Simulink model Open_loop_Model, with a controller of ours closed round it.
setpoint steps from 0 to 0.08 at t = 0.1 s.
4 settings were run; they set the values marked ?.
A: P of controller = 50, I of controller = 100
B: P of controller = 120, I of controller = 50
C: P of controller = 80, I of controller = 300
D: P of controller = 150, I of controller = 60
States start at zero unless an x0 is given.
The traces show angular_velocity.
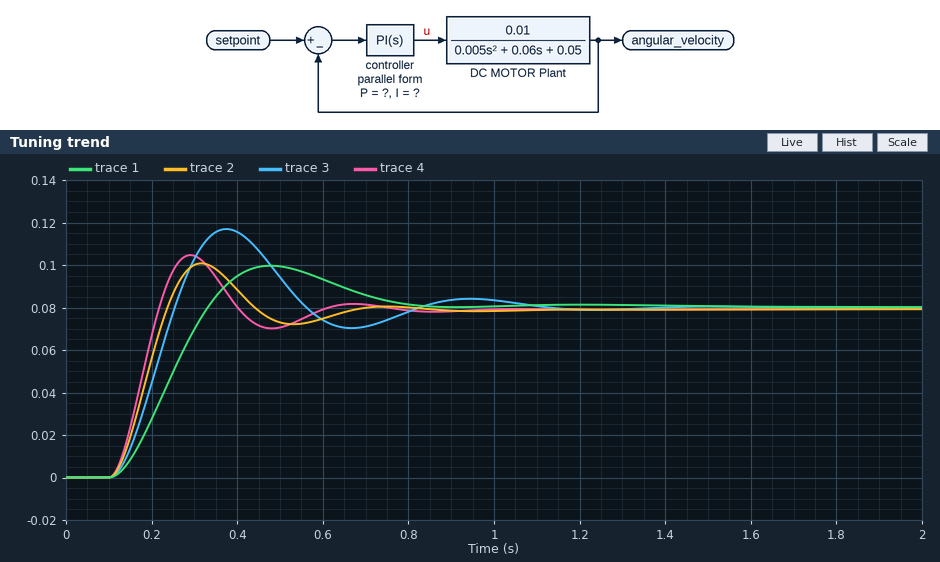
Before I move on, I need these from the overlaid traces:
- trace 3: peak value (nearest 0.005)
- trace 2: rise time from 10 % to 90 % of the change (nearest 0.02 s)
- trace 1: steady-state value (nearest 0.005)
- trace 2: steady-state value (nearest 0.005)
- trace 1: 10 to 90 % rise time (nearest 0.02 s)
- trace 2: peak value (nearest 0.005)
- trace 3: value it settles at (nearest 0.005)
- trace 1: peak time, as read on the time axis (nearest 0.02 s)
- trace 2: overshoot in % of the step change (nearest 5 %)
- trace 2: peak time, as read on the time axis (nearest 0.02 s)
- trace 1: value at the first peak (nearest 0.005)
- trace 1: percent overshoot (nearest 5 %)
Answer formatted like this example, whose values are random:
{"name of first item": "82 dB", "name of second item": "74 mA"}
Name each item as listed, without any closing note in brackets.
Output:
{"trace 3: peak value": "0.115", "trace 2: rise time from 10 % to 90 % of the change": "0.10 s", "trace 1: steady-state value": "0.080", "trace 2: steady-state value": "0.080", "trace 1: 10 to 90 % rise time": "0.16 s", "trace 2: peak value": "0.100", "trace 3: value it settles at": "0.080", "trace 1: peak time, as read on the time axis": "0.48 s", "trace 2: overshoot in % of the step change": "25 %", "trace 2: peak time, as read on the time axis": "0.32 s", "trace 1: value at the first peak": "0.100", "trace 1: percent overshoot": "25 %"}
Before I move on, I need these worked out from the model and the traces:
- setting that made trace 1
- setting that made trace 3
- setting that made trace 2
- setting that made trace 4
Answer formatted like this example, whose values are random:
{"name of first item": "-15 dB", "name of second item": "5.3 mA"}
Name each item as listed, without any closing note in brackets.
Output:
{"setting that made trace 1": "A", "setting that made trace 3": "C", "setting that made trace 2": "B", "setting that made trace 4": "D"}
